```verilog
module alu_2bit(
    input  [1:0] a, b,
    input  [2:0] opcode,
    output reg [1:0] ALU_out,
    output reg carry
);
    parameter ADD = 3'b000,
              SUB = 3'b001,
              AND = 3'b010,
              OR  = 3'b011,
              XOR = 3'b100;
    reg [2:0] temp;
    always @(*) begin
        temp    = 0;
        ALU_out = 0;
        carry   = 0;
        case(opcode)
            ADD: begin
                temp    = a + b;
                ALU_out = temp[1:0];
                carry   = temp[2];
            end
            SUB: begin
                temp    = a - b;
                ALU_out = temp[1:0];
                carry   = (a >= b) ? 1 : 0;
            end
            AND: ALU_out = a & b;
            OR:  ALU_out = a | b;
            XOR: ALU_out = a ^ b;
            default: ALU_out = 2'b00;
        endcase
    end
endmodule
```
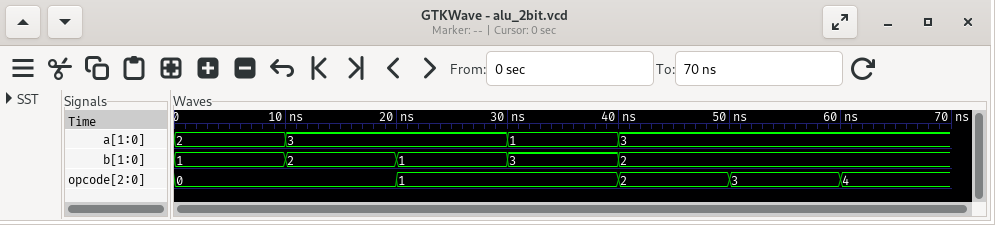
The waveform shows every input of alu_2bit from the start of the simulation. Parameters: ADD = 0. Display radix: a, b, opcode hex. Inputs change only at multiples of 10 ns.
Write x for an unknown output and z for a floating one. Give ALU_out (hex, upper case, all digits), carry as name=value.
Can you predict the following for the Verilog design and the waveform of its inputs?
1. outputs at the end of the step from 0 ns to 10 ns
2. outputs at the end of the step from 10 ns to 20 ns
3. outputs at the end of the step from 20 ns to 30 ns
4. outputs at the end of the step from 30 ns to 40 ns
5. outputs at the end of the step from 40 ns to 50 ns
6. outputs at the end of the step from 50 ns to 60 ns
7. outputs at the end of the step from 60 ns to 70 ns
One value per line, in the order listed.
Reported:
ALU_out=3, carry=0
ALU_out=1, carry=1
ALU_out=2, carry=1
ALU_out=2, carry=0
ALU_out=2, carry=0
ALU_out=3, carry=0
ALU_out=1, carry=0
